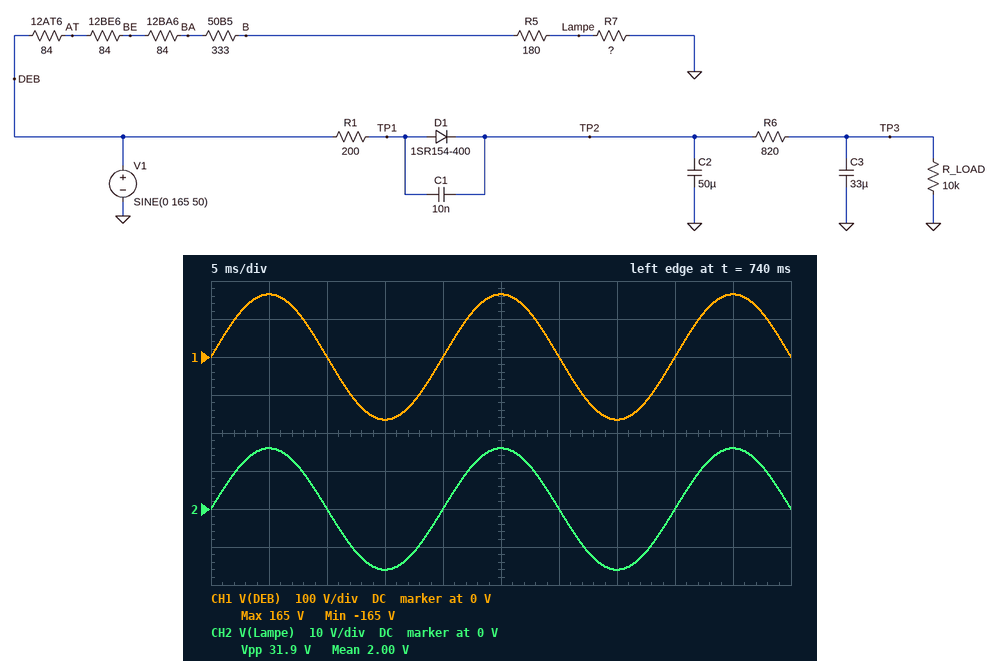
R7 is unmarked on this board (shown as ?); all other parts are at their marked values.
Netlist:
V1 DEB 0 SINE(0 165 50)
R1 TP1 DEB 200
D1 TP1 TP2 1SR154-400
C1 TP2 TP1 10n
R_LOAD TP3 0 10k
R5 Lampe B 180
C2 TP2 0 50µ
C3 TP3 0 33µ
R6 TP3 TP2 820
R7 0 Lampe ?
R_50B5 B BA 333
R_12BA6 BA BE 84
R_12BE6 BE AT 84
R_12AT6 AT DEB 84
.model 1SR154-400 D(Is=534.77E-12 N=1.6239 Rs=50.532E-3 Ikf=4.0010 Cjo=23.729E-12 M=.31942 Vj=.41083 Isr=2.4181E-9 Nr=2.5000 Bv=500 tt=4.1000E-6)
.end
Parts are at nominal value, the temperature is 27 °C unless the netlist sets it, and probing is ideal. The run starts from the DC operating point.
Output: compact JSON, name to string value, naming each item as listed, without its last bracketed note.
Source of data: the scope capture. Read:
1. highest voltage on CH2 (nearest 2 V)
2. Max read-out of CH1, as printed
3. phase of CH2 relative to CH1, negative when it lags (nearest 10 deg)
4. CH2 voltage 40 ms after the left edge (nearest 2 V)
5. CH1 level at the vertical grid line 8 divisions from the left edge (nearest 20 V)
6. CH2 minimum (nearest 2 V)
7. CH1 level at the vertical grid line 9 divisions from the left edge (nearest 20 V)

{"highest voltage on CH2": "16 V", "Max read-out of CH1, as printed": "165 V", "phase of CH2 relative to CH1, negative when it lags": "0 deg", "CH2 voltage 40 ms after the left edge": "0 V", "CH1 level at the vertical grid line 8 divisions from the left edge": "0 V", "CH2 minimum": "-16 V", "CH1 level at the vertical grid line 9 divisions from the left edge": "160 V"}
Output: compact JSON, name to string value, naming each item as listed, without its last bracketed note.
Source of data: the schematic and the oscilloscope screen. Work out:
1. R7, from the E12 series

{"R7, from the E12 series": "82 Ω"}
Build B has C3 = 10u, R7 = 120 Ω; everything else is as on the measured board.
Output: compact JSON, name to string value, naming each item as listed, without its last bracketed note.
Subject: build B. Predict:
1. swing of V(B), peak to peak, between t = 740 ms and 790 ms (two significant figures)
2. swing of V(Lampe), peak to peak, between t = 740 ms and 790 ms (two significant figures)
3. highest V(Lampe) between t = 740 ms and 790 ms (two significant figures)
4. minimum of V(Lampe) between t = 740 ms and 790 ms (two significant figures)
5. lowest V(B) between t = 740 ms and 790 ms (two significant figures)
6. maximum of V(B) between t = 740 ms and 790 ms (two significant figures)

{"swing of V(B), peak to peak, between t = 740 ms and 790 ms": "110 V", "swing of V(Lampe), peak to peak, between t = 740 ms and 790 ms": "45 V", "highest V(Lampe) between t = 740 ms and 790 ms": "22 V", "minimum of V(Lampe) between t = 740 ms and 790 ms": "-22 V", "lowest V(B) between t = 740 ms and 790 ms": "-56 V", "maximum of V(B) between t = 740 ms and 790 ms": "56 V"}
